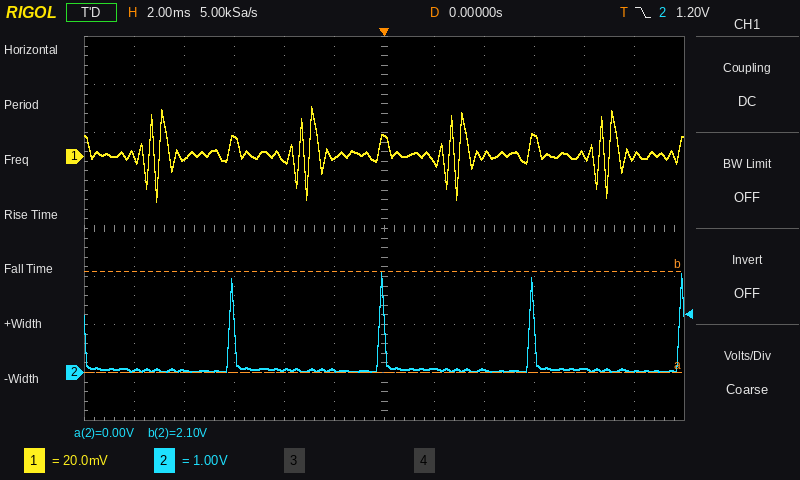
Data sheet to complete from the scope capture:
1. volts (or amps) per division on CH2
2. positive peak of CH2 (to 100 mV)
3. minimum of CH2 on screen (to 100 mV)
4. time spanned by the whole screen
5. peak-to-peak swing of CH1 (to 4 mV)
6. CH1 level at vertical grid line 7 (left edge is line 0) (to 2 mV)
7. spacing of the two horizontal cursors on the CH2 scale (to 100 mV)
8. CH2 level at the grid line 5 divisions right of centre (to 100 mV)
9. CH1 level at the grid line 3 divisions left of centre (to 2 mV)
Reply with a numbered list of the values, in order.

1. 1 V
2. 2.1 V
3. 0.0 V
4. 24 ms
5. 40 mV
6. -2 mV
7. 2.1 V
8. 0.0 V
9. 8 mV
